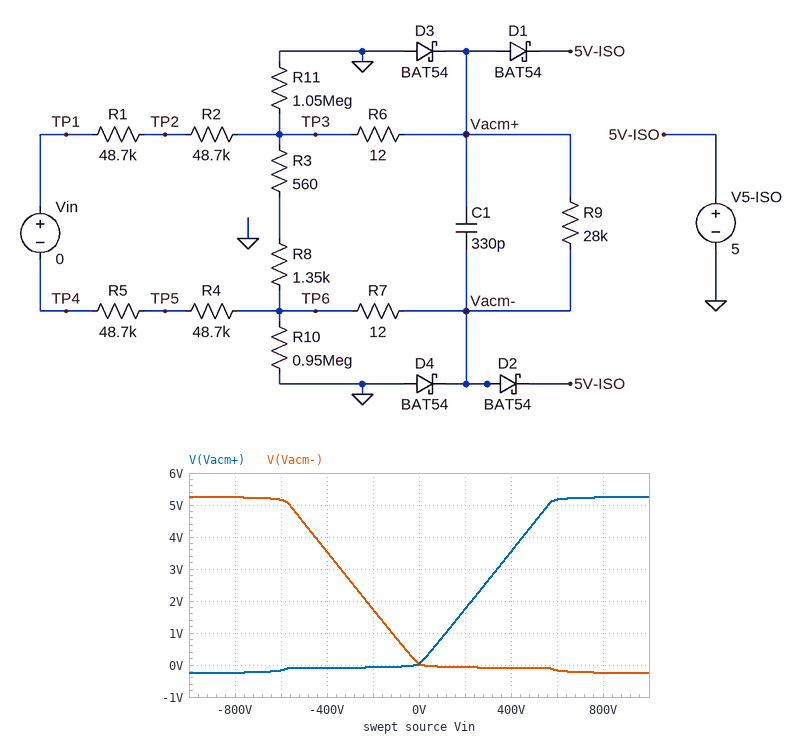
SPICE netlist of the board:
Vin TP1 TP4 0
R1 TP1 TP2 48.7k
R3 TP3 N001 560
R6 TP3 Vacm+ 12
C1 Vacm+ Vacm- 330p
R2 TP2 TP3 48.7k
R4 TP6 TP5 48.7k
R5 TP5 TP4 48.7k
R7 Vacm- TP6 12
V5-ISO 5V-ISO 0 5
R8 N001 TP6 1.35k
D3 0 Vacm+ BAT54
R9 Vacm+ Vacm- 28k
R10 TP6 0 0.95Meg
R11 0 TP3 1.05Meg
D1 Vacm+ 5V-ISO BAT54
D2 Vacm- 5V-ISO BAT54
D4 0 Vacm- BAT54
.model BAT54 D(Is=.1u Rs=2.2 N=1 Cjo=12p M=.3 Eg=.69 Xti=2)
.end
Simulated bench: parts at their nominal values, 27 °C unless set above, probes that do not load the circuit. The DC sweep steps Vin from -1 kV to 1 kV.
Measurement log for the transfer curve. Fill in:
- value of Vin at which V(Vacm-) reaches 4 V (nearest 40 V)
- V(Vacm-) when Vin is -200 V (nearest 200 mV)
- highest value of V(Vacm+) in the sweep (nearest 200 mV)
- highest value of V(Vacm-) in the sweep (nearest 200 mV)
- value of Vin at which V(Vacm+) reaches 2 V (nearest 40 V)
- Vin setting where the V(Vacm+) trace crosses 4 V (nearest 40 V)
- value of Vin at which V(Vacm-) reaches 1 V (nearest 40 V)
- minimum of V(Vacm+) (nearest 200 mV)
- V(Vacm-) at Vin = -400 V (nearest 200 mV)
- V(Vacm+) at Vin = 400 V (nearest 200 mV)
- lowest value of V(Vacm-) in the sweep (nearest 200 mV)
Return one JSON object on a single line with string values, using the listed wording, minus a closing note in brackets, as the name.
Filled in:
{"value of Vin at which V(Vacm-) reaches 4 V": "-440 V", "V(Vacm-) when Vin is -200 V": "1.8 V", "highest value of V(Vacm+) in the sweep": "5.2 V", "highest value of V(Vacm-) in the sweep": "5.2 V", "value of Vin at which V(Vacm+) reaches 2 V": "240 V", "Vin setting where the V(Vacm+) trace crosses 4 V": "440 V", "value of Vin at which V(Vacm-) reaches 1 V": "-120 V", "minimum of V(Vacm+)": "-200 mV", "V(Vacm-) at Vin = -400 V": "3.6 V", "V(Vacm+) at Vin = 400 V": "3.6 V", "lowest value of V(Vacm-) in the sweep": "-200 mV"}
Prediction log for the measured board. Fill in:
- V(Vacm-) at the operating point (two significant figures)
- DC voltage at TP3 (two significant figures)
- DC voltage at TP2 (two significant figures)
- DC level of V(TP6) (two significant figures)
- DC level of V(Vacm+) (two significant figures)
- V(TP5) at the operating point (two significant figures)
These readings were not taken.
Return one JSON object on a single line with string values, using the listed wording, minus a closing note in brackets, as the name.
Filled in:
{"V(Vacm-) at the operating point": "31 mV", "DC voltage at TP3": "31 mV", "DC voltage at TP2": "31 mV", "DC level of V(TP6)": "31 mV", "DC level of V(Vacm+)": "31 mV", "V(TP5) at the operating point": "31 mV"}
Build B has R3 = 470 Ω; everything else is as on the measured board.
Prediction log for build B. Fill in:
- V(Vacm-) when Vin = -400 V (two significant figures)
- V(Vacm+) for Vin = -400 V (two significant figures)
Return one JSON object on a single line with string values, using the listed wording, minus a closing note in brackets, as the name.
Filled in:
{"V(Vacm-) when Vin = -400 V": "3.4 V", "V(Vacm+) for Vin = -400 V": "-92 mV"}
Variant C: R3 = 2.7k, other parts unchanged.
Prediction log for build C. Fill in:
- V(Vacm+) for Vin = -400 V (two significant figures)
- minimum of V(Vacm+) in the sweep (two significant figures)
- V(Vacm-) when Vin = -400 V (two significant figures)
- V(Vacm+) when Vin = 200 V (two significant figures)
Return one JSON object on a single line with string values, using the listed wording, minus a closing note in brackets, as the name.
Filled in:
{"V(Vacm+) for Vin = -400 V": "-220 mV", "minimum of V(Vacm+) in the sweep": "-280 mV", "V(Vacm-) when Vin = -400 V": "5.2 V", "V(Vacm+) when Vin = 200 V": "3.5 V"}
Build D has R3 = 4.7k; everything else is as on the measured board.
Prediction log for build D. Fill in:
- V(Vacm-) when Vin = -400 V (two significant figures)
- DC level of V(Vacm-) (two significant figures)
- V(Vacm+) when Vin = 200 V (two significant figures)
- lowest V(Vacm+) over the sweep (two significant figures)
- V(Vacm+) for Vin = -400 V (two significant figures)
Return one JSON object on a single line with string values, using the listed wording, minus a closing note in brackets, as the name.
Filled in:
{"V(Vacm-) when Vin = -400 V": "5.2 V", "DC level of V(Vacm-)": "31 mV", "V(Vacm+) when Vin = 200 V": "4.9 V", "lowest V(Vacm+) over the sweep": "-280 mV", "V(Vacm+) for Vin = -400 V": "-240 mV"}
